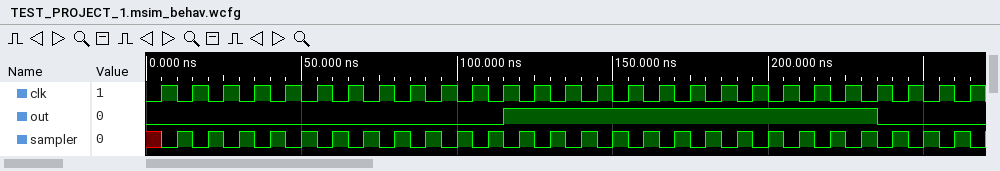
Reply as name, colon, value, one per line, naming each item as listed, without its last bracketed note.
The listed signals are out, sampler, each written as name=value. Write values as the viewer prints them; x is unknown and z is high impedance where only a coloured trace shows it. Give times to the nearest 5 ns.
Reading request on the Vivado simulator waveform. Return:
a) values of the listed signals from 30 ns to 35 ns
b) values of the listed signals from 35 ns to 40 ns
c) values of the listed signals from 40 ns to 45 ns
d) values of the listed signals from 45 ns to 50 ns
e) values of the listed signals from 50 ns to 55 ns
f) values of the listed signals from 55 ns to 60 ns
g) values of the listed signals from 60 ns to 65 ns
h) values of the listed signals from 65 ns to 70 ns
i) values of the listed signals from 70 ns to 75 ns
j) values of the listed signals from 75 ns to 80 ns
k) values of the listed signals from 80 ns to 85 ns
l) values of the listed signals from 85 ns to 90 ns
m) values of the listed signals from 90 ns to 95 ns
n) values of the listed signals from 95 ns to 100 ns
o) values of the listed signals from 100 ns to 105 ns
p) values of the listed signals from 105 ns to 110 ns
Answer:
values of the listed signals from 30 ns to 35 ns: out=0, sampler=1
values of the listed signals from 35 ns to 40 ns: out=0, sampler=0
values of the listed signals from 40 ns to 45 ns: out=0, sampler=1
values of the listed signals from 45 ns to 50 ns: out=0, sampler=0
values of the listed signals from 50 ns to 55 ns: out=0, sampler=1
values of the listed signals from 55 ns to 60 ns: out=0, sampler=0
values of the listed signals from 60 ns to 65 ns: out=0, sampler=1
values of the listed signals from 65 ns to 70 ns: out=0, sampler=0
values of the listed signals from 70 ns to 75 ns: out=0, sampler=1
values of the listed signals from 75 ns to 80 ns: out=0, sampler=0
values of the listed signals from 80 ns to 85 ns: out=0, sampler=1
values of the listed signals from 85 ns to 90 ns: out=0, sampler=0
values of the listed signals from 90 ns to 95 ns: out=0, sampler=1
values of the listed signals from 95 ns to 100 ns: out=0, sampler=0
values of the listed signals from 100 ns to 105 ns: out=0, sampler=1
values of the listed signals from 105 ns to 110 ns: out=0, sampler=0
